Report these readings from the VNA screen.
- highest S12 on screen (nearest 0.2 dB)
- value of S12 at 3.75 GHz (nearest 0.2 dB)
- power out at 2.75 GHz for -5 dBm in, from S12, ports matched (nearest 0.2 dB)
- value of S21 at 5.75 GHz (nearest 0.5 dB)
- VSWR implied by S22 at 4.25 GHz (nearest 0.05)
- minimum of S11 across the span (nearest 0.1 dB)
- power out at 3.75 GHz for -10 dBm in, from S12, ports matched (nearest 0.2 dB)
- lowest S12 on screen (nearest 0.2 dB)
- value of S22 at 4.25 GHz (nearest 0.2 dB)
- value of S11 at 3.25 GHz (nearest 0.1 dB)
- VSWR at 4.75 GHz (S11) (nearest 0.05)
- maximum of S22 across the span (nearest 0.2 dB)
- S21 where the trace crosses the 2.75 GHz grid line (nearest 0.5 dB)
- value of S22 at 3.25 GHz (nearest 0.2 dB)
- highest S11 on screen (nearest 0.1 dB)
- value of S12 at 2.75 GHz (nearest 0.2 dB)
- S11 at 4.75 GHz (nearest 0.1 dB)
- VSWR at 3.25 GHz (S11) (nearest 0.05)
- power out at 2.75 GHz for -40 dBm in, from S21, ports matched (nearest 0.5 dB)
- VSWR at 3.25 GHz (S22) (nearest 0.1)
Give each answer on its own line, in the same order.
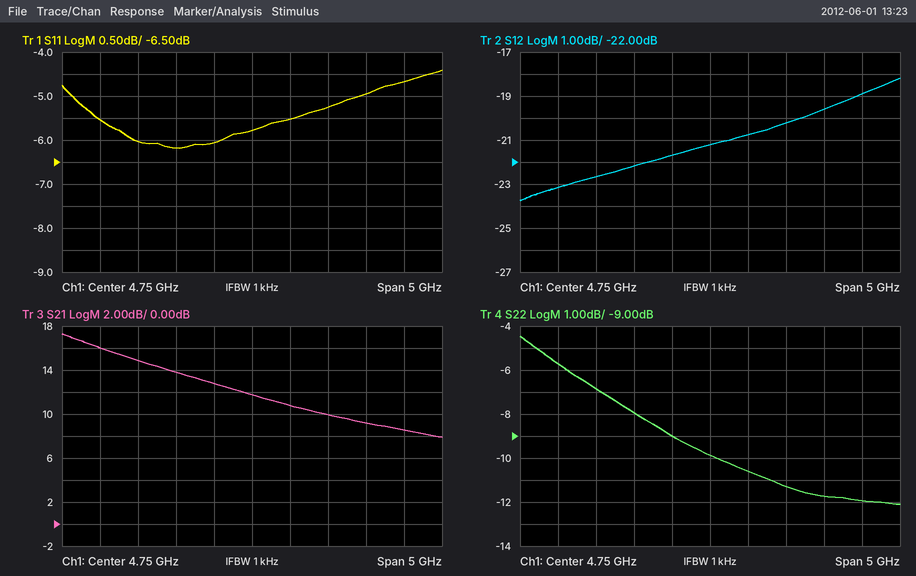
-18.2 dB
-22.2 dB
-28.2 dBm
10.0 dB
2.10
-6.2 dB
-32.2 dBm
-23.8 dB
-9.0 dB
-6.0 dB
3.10
-4.4 dB
16.0 dB
-6.8 dB
-4.4 dB
-23.2 dB
-5.8 dB
3.00
-24.0 dBm
2.7
